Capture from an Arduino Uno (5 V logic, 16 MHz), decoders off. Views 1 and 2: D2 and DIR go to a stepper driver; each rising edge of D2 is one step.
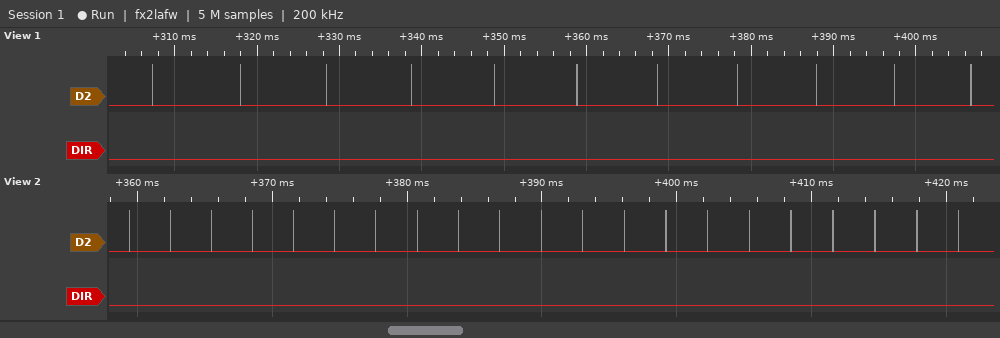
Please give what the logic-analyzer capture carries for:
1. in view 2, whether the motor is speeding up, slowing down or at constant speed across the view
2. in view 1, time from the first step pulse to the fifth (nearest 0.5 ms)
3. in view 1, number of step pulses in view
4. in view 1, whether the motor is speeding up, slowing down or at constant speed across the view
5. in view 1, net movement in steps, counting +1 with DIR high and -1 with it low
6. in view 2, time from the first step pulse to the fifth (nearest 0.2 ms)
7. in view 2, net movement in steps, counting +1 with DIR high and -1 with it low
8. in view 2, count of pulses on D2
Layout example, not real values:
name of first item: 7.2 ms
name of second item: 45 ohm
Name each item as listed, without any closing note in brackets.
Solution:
in view 2, whether the motor is speeding up, slowing down or at constant speed across the view: constant speed
in view 1, time from the first step pulse to the fifth: 41.5 ms
in view 1, number of step pulses in view: 11
in view 1, whether the motor is speeding up, slowing down or at constant speed across the view: speeding up
in view 1, net movement in steps, counting +1 with DIR high and -1 with it low: -11
in view 2, time from the first step pulse to the fifth: 12.2 ms
in view 2, net movement in steps, counting +1 with DIR high and -1 with it low: -21
in view 2, count of pulses on D2: 21
